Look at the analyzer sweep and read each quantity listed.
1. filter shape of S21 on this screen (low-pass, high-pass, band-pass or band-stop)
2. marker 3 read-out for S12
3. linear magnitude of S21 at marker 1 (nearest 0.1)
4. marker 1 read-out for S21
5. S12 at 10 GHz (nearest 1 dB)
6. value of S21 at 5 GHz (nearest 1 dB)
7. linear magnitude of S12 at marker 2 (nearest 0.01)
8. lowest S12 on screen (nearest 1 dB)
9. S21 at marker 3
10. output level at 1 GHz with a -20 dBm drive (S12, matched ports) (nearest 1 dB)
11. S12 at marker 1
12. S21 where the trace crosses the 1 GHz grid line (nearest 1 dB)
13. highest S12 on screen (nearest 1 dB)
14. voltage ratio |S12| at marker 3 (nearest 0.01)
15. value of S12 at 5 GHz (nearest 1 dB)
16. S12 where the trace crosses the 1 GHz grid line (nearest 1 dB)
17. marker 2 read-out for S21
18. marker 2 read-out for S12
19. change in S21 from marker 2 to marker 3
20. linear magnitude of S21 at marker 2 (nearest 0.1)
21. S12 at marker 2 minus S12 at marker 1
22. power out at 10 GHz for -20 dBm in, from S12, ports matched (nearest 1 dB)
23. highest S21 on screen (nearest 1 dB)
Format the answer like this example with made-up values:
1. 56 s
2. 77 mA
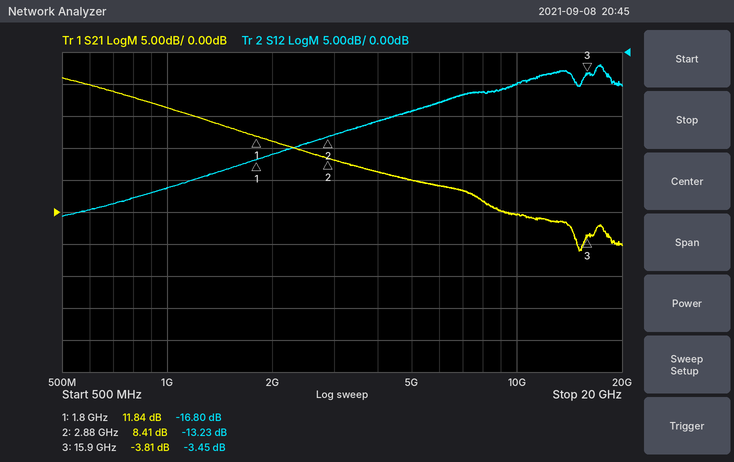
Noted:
1. low-pass
2. -3.45 dB
3. 3.9
4. 11.84 dB
5. -5 dB
6. 5 dB
7. 0.22
8. -26 dB
9. -3.81 dB
10. -41 dBm
11. -16.80 dB
12. 16 dB
13. -2 dB
14. 0.67
15. -9 dB
16. -21 dB
17. 8.41 dB
18. -13.23 dB
19. -12.22 dB
20. 2.6
21. 3.57 dB
22. -25 dBm
23. 21 dB
